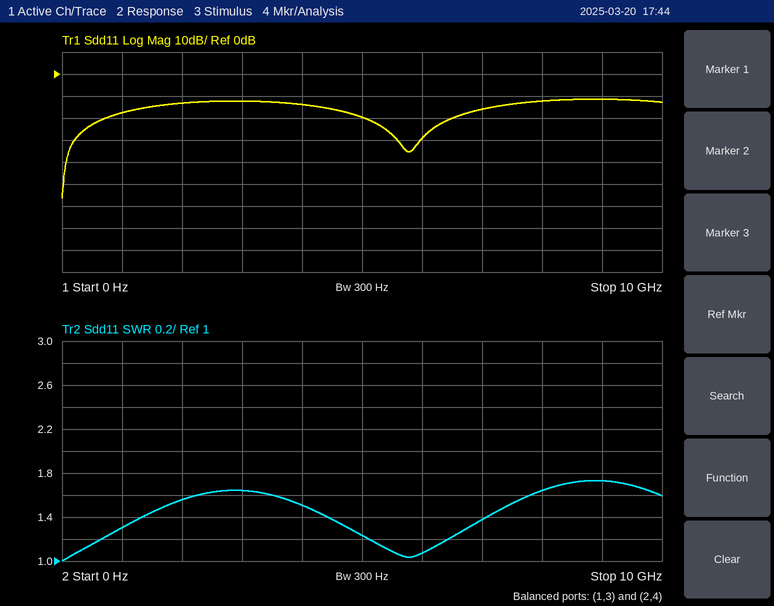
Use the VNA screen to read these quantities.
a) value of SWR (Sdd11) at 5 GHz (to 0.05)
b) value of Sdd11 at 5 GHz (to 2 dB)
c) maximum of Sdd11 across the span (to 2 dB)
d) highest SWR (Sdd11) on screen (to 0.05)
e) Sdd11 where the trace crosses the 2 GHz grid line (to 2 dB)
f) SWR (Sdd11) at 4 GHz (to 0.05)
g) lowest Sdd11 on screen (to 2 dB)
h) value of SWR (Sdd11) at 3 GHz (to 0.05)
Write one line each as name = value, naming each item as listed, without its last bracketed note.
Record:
value of SWR (Sdd11) at 5 GHz = 1.25
value of Sdd11 at 5 GHz = -20 dB
maximum of Sdd11 across the span = -12 dB
highest SWR (Sdd11) on screen = 1.75
Sdd11 where the trace crosses the 2 GHz grid line = -14 dB
SWR (Sdd11) at 4 GHz = 1.50
lowest Sdd11 on screen = -56 dB
value of SWR (Sdd11) at 3 GHz = 1.65
